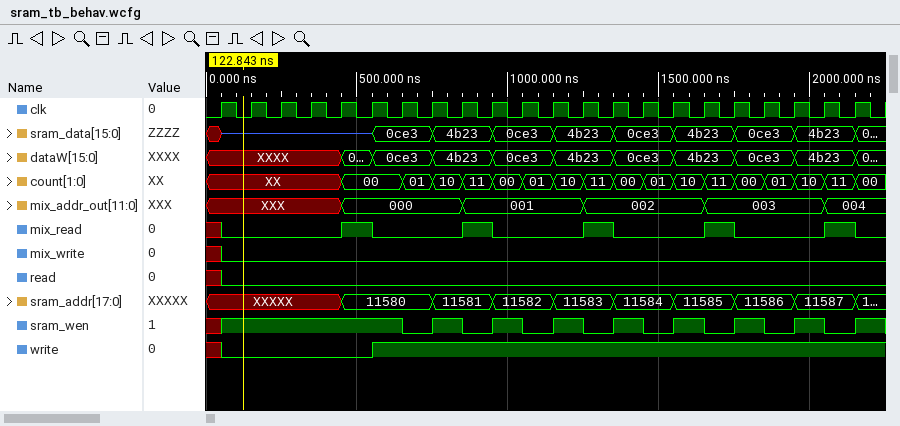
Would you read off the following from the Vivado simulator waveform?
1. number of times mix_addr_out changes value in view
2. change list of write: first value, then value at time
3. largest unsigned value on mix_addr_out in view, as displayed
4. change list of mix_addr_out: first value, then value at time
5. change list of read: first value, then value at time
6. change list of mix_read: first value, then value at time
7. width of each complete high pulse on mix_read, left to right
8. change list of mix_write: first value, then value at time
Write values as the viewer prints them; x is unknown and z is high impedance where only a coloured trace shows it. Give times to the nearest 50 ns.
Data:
5
x, 0 at 50 ns, 1 at 550 ns
004
XXX, 000 at 450 ns, 001 at 850 ns, 002 at 1250 ns, 003 at 1650 ns, 004 at 2050 ns
x, 0 at 50 ns
x, 0 at 50 ns, 1 at 450 ns, 0 at 550 ns, 1 at 850 ns, 0 at 950 ns, 1 at 1250 ns, 0 at 1350 ns, 1 at 1650 ns, 0 at 1750 ns, 1 at 2050 ns, 0 at 2150 ns
100 ns, 100 ns, 100 ns, 100 ns, 100 ns
x, 0 at 50 ns
